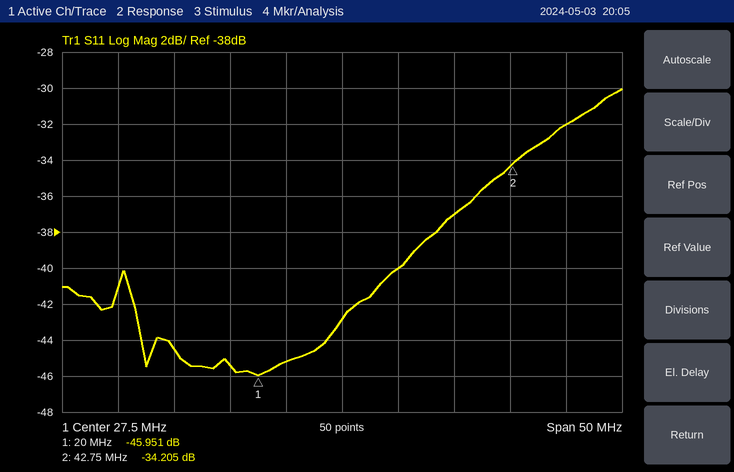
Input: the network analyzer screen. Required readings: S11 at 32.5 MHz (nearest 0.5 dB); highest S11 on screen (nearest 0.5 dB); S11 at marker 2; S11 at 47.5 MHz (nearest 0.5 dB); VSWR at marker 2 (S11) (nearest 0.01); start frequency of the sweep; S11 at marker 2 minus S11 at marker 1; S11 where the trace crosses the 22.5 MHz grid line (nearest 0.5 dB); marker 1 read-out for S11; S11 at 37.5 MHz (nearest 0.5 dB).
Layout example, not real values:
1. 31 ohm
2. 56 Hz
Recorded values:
1. -40.0 dB
2. -30.0 dB
3. -34.205 dB
4. -32.0 dB
5. 1.04
6. 2.5 MHz
7. 11.746 dB
8. -45.0 dB
9. -45.951 dB
10. -37.0 dB
